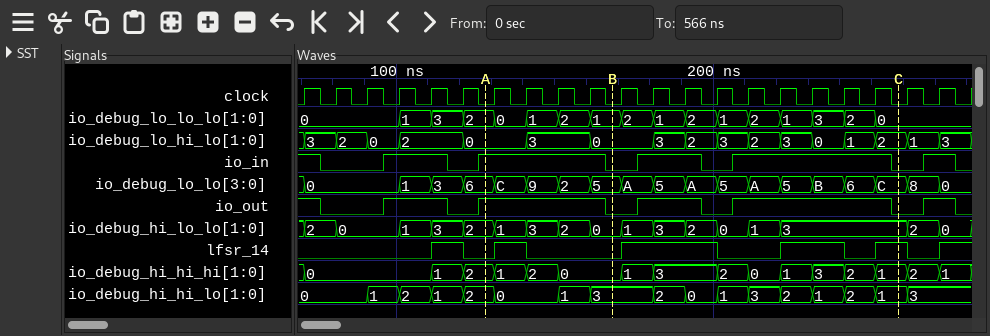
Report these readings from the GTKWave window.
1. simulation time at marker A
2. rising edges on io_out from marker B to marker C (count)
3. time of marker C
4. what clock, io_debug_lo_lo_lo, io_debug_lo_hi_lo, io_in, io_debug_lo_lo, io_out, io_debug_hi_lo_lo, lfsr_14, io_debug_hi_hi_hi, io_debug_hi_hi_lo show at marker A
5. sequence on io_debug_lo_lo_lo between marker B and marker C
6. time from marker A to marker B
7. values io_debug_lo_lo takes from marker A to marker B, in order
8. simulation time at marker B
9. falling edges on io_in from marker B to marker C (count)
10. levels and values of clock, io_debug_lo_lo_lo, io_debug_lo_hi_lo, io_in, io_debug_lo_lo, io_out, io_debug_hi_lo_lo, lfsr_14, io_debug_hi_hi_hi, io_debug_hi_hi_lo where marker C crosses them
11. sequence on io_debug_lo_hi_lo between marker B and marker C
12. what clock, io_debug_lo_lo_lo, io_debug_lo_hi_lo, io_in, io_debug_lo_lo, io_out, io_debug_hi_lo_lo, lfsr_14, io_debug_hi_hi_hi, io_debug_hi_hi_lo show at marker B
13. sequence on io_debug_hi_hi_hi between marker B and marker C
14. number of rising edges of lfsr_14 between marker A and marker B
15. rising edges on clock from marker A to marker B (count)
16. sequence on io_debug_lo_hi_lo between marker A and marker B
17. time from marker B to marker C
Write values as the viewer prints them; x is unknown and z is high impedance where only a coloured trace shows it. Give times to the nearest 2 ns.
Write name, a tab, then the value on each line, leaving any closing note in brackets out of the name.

simulation time at marker A	128 ns
rising edges on io_out from marker B to marker C	2
time of marker C	258 ns
what clock, io_debug_lo_lo_lo, io_debug_lo_hi_lo, io_in, io_debug_lo_lo, io_out, io_debug_hi_lo_lo, lfsr_14, io_debug_hi_hi_hi, io_debug_hi_hi_lo show at marker A	clock=0, io_debug_lo_lo_lo=2, io_debug_lo_hi_lo=0, io_in=1, io_debug_lo_lo=6, io_out=1, io_debug_hi_lo_lo=2, lfsr_14=0, io_debug_hi_hi_hi=2, io_debug_hi_hi_lo=2
sequence on io_debug_lo_lo_lo between marker B and marker C	1, 2, 1, 2, 1, 2, 1, 3, 2, 0
time from marker A to marker B	40 ns
values io_debug_lo_lo takes from marker A to marker B, in order	6, C, 9, 2, 5
simulation time at marker B	168 ns
falling edges on io_in from marker B to marker C	2
levels and values of clock, io_debug_lo_lo_lo, io_debug_lo_hi_lo, io_in, io_debug_lo_lo, io_out, io_debug_hi_lo_lo, lfsr_14, io_debug_hi_hi_hi, io_debug_hi_hi_lo where marker C crosses them	clock=0, io_debug_lo_lo_lo=0, io_debug_lo_hi_lo=2, io_in=0, io_debug_lo_lo=C, io_out=0, io_debug_hi_lo_lo=3, lfsr_14=1, io_debug_hi_hi_hi=1, io_debug_hi_hi_lo=1
sequence on io_debug_lo_hi_lo between marker B and marker C	0, 3, 2, 3, 2, 3, 0, 1, 2
what clock, io_debug_lo_lo_lo, io_debug_lo_hi_lo, io_in, io_debug_lo_lo, io_out, io_debug_hi_lo_lo, lfsr_14, io_debug_hi_hi_hi, io_debug_hi_hi_lo show at marker B	clock=0, io_debug_lo_lo_lo=1, io_debug_lo_hi_lo=0, io_in=0, io_debug_lo_lo=5, io_out=0, io_debug_hi_lo_lo=0, lfsr_14=0, io_debug_hi_hi_hi=0, io_debug_hi_hi_lo=3
sequence on io_debug_hi_hi_hi between marker B and marker C	0, 1, 3, 2, 0, 1, 3, 2, 1
number of rising edges of lfsr_14 between marker A and marker B	1
rising edges on clock from marker A to marker B	4
sequence on io_debug_lo_hi_lo between marker A and marker B	0, 3, 0
time from marker B to marker C	90 ns
